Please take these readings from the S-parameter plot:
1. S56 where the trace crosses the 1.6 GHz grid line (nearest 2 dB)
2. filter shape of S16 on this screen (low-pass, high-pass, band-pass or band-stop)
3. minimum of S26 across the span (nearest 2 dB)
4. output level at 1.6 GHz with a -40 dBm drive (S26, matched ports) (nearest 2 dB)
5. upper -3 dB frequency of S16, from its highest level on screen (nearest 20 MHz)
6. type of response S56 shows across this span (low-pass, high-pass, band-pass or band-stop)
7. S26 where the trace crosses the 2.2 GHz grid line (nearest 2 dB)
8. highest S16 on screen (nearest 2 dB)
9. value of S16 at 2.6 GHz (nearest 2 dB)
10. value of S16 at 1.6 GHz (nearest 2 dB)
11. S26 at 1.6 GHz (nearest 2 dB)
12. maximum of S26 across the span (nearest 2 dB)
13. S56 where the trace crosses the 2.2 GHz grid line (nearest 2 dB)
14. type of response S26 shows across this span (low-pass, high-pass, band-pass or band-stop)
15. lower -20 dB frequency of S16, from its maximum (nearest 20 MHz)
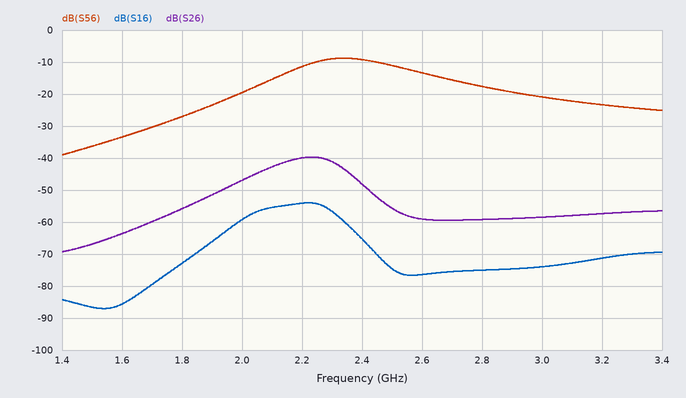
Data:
-34 dB
band-pass
-70 dB
-104 dBm
2.30 GHz
band-pass
-40 dB
-54 dB
-76 dB
-86 dB
-64 dB
-40 dB
-12 dB
band-pass
1.78 GHz
